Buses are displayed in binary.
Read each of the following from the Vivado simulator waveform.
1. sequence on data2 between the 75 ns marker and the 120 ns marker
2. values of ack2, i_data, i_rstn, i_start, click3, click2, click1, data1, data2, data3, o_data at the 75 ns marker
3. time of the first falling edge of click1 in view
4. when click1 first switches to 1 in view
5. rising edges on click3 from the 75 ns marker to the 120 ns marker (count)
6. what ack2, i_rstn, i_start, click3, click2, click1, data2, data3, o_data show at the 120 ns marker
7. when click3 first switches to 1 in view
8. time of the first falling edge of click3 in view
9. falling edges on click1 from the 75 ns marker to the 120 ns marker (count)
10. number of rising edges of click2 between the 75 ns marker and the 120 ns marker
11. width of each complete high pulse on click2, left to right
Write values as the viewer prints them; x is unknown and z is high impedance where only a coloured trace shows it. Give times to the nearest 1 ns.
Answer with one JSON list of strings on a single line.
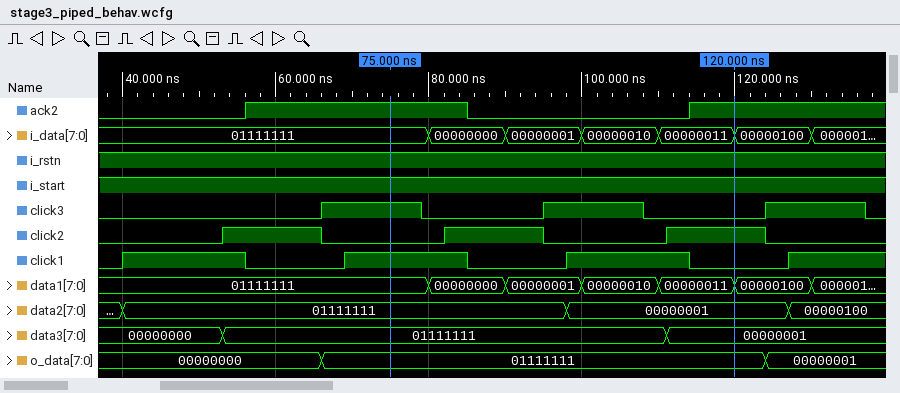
["01111111, 00000001", "ack2=1, i_data=01111111, i_rstn=1, i_start=1, click3=1, click2=0, click1=1, data1=01111111, data2=01111111, data3=01111111, o_data=01111111", "56 ns", "40 ns", "1", "ack2=1, i_rstn=1, i_start=1, click3=0, click2=1, click1=0, data2=00000001, data3=00000001, o_data=01111111", "66 ns", "79 ns", "2", "2", "13 ns, 13 ns, 13 ns"]
